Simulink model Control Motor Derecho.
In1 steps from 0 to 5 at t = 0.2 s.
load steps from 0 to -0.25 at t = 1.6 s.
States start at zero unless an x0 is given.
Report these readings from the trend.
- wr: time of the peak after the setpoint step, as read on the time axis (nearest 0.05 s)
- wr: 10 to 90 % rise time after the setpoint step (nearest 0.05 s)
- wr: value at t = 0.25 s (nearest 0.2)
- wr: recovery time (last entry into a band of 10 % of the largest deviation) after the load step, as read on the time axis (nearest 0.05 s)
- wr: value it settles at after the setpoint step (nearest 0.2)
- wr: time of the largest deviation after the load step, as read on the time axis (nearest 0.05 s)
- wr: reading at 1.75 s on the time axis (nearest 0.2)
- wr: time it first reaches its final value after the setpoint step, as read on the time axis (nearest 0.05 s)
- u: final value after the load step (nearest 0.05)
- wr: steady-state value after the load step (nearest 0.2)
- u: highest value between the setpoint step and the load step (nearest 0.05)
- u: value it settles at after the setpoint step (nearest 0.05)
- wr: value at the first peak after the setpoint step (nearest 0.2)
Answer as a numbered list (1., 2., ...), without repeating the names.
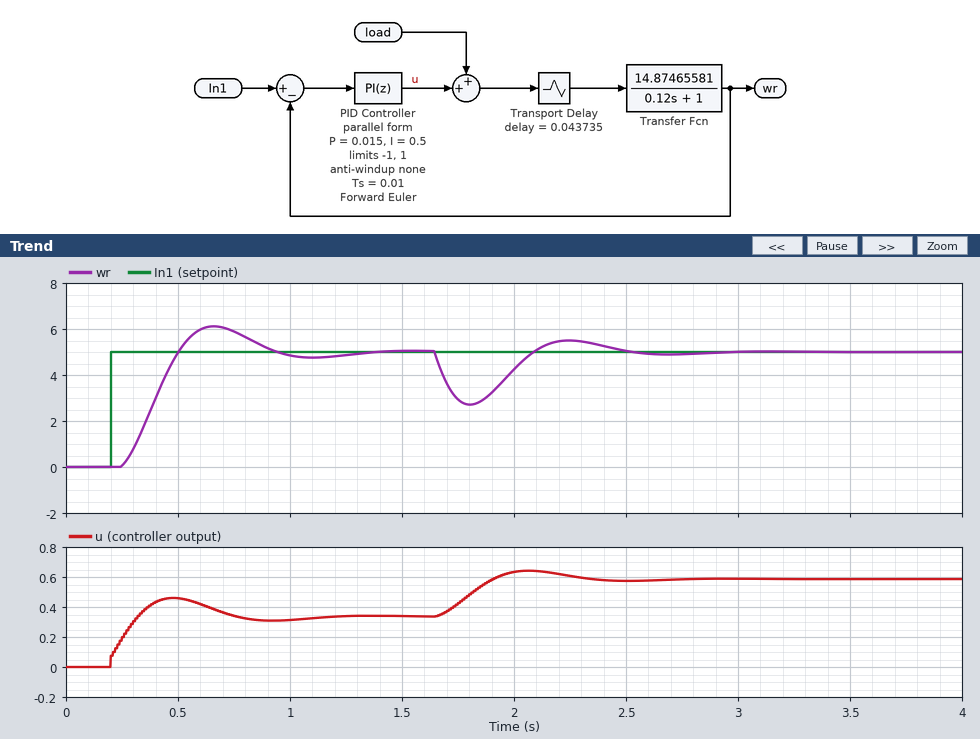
1. 0.65 s
2. 0.20 s
3. 0.0
4. 2.40 s
5. 5.0
6. 1.80 s
7. 3.0
8. 0.50 s
9. 0.60
10. 5.0
11. 0.45
12. 0.35
13. 6.2
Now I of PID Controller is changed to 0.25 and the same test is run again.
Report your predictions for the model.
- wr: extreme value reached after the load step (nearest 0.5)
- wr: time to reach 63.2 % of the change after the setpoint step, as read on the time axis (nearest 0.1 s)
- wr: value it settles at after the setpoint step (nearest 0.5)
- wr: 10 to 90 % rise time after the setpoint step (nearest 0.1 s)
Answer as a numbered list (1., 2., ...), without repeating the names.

1. 2.5
2. 0.5 s
3. 5.0
4. 0.4 s
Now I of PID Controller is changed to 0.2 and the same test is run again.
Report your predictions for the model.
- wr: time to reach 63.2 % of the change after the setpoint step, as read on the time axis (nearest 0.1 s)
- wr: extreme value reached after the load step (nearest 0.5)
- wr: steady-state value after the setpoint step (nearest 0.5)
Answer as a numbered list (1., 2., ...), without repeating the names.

1. 0.6 s
2. 2.5
3. 5.0
